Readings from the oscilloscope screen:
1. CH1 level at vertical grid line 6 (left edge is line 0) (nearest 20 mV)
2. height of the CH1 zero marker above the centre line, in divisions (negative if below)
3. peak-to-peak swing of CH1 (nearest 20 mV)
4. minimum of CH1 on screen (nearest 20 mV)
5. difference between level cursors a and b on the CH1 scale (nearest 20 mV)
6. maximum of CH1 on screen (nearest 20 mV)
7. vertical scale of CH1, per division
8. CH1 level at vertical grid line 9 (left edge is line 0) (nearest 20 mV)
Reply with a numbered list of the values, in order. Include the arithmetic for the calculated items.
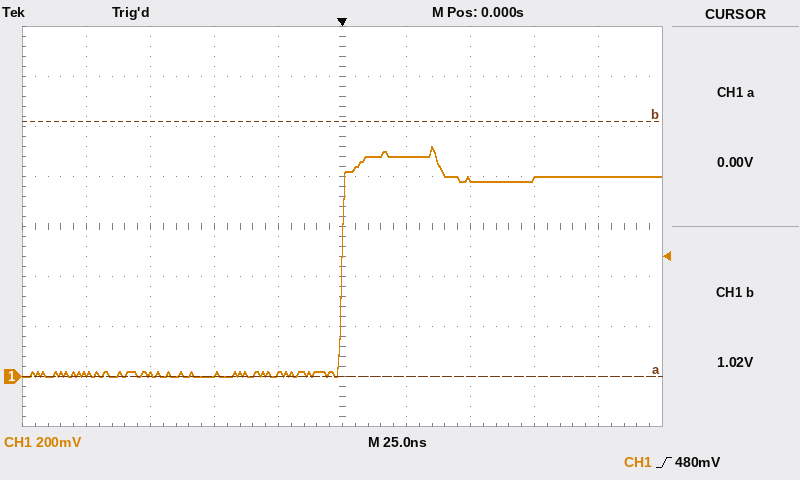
1. 880 mV
2. -3.0 div
3. 920 mV − (0 mV) = 920 mV
4. 0 mV
5. 1.02 V
6. 920 mV
7. 200 mV
8. 800 mV
